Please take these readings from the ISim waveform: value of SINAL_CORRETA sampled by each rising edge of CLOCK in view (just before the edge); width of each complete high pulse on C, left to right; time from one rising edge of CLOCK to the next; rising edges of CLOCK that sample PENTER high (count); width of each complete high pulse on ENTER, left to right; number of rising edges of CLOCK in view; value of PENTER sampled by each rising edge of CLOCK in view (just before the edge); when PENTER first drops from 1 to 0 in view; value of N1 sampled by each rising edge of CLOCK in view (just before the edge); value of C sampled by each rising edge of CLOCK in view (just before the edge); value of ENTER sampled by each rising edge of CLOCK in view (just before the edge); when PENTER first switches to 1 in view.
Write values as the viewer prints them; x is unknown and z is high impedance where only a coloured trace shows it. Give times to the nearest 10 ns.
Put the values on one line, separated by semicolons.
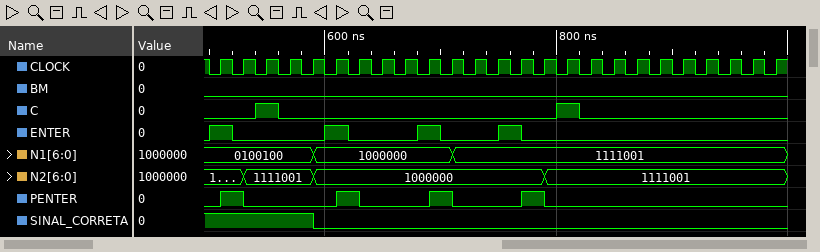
1 1 1 1 1 0 0 0 0 0 0 0 0 0 0 0 0 0 0 0 0 0 0 0 0; 20 ns, 20 ns; 20 ns; 4; 20 ns, 20 ns, 20 ns, 20 ns; 25; 0 1 0 0 0 0 1 0 0 0 1 0 0 0 1 0 0 0 0 0 0 0 0 0 0; 530 ns; 0100100, 0100100, 0100100, 0100100, 0100100, 1000000, 1000000, 1000000, 1000000, 1000000, 1000000, 1111001, 1111001, 1111001, 1111001, 1111001, 1111001, 1111001, 1111001, 1111001, 1111001, 1111001, 1111001, 1111001, 1111001; 0 0 1 0 0 0 0 0 0 0 0 0 0 0 0 1 0 0 0 0 0 0 0 0 0; 1 0 0 0 0 1 0 0 0 1 0 0 0 1 0 0 0 0 0 0 0 0 0 0 0; 510 ns
